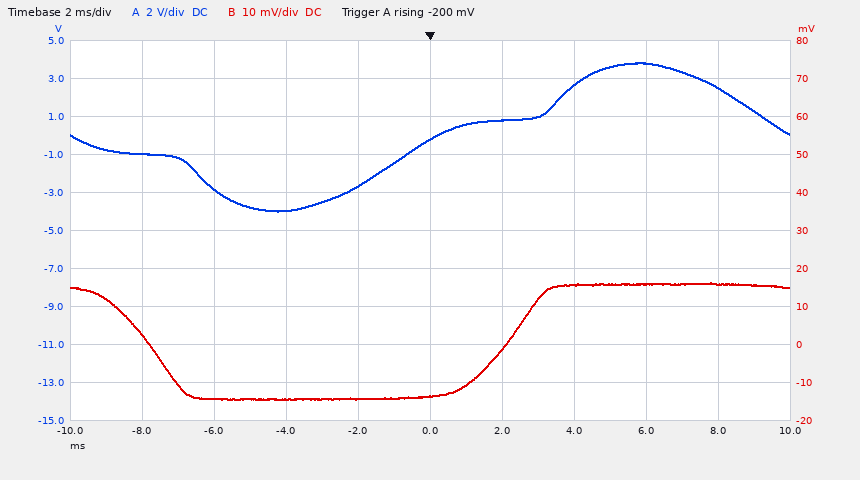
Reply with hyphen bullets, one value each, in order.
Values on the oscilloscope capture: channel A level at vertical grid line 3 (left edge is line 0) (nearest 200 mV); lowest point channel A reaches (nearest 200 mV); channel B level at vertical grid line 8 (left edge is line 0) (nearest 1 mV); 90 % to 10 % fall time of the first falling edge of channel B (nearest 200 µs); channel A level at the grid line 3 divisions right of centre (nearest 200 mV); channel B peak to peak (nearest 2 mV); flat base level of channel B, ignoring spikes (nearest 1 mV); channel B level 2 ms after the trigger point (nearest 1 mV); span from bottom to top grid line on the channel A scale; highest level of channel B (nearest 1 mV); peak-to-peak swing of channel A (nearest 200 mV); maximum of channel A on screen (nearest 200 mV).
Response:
- -4.0 V
- -4.0 V
- 16 mV
- 2.2 ms
- 3.8 V
- 30 mV
- -14 mV
- -1 mV
- 20 V
- 16 mV
- 7.8 V
- 3.8 V
